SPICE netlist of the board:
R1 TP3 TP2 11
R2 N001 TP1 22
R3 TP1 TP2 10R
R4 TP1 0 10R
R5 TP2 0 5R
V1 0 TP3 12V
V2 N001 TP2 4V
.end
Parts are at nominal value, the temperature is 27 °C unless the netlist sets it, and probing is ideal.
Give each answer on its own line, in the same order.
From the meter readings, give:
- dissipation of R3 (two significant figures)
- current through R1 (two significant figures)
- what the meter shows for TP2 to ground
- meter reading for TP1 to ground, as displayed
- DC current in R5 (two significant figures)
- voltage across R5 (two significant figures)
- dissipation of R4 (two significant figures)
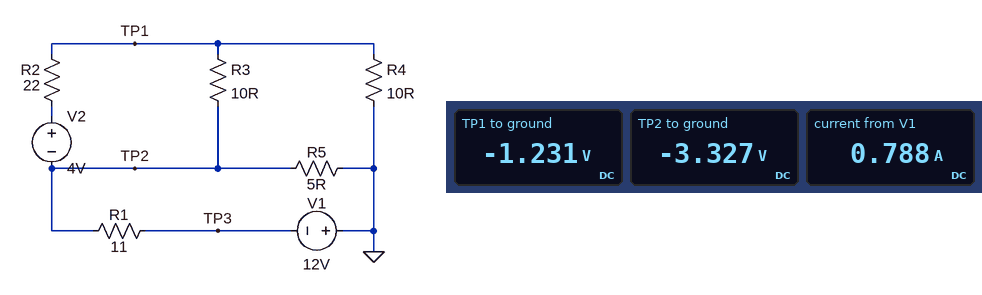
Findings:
440 mW
790 mA
-3.327 V
-1.231 V
670 mA
3.3 V
150 mW
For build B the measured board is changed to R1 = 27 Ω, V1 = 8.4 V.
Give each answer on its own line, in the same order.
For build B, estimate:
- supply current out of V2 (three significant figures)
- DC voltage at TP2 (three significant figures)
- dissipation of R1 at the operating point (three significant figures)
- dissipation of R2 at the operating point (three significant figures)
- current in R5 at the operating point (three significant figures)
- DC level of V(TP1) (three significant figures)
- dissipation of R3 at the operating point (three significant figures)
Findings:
124 mA
-1.30 V
1.87 W
339 mW
260 mA
-29.6 mV
161 mW
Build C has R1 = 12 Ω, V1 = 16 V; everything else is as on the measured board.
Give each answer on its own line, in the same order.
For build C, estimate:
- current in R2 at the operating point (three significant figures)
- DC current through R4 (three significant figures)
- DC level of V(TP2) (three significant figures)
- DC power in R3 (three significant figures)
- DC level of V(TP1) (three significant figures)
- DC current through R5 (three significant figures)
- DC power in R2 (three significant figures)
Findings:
72.1 mA
169 mA
-4.11 V
583 mW
-1.69 V
822 mA
114 mW
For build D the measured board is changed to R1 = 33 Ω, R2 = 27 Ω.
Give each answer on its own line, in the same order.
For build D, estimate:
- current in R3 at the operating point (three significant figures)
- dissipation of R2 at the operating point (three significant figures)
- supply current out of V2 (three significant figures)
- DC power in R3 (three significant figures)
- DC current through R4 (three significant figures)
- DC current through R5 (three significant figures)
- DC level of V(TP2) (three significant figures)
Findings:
125 mA
280 mW
102 mA
156 mW
23.0 mA
296 mA
-1.48 V
